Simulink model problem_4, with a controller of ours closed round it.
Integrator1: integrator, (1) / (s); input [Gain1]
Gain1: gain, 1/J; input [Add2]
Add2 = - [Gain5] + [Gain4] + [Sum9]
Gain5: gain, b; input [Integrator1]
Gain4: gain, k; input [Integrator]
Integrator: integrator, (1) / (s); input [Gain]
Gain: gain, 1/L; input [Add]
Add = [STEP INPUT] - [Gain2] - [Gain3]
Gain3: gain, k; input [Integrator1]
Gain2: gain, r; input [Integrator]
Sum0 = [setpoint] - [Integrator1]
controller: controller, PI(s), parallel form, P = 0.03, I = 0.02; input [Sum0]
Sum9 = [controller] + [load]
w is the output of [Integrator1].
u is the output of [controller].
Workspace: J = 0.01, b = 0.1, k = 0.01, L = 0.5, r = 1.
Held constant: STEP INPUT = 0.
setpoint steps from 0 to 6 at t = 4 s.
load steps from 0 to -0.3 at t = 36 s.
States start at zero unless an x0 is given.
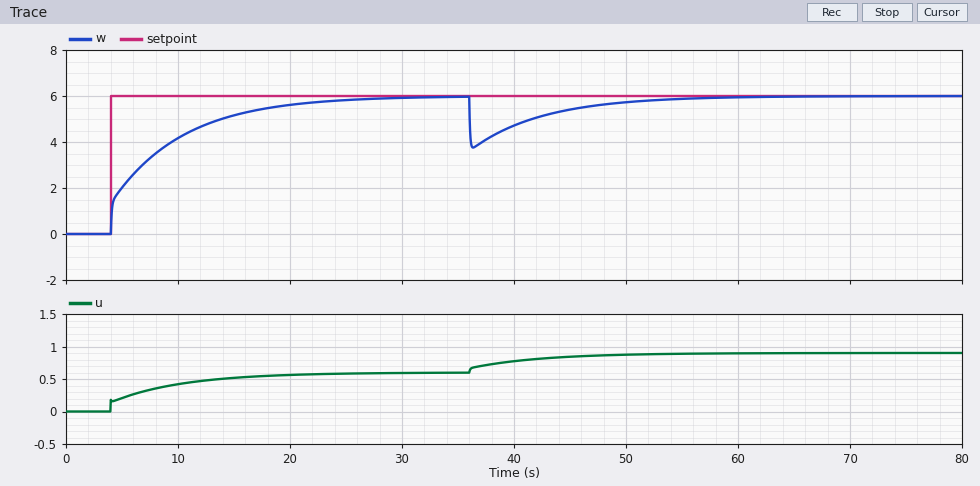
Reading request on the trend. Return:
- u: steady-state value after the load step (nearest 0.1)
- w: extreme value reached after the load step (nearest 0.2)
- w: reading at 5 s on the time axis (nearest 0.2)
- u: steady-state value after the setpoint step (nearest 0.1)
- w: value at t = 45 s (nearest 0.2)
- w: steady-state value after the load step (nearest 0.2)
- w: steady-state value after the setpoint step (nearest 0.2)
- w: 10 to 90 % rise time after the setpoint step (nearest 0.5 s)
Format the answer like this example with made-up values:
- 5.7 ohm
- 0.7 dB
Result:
- 0.9
- 3.8
- 2.0
- 0.6
- 5.4
- 6.0
- 6.0
- 13.0 s
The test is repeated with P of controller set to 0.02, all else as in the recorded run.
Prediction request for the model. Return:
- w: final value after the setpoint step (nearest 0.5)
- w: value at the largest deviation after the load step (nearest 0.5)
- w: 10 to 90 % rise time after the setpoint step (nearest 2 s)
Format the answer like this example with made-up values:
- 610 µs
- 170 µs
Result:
- 6.0
- 3.5
- 12 s
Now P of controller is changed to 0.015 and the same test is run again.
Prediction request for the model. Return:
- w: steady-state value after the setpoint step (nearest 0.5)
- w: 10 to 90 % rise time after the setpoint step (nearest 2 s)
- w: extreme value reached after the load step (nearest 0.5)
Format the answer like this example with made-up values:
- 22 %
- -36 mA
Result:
- 6.0
- 12 s
- 3.5
